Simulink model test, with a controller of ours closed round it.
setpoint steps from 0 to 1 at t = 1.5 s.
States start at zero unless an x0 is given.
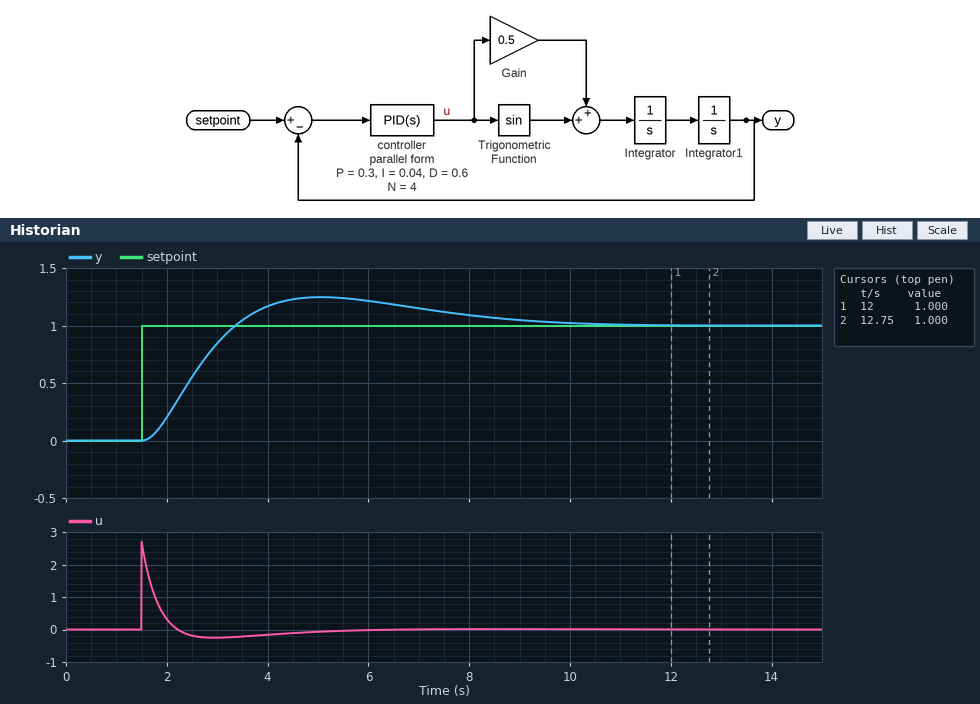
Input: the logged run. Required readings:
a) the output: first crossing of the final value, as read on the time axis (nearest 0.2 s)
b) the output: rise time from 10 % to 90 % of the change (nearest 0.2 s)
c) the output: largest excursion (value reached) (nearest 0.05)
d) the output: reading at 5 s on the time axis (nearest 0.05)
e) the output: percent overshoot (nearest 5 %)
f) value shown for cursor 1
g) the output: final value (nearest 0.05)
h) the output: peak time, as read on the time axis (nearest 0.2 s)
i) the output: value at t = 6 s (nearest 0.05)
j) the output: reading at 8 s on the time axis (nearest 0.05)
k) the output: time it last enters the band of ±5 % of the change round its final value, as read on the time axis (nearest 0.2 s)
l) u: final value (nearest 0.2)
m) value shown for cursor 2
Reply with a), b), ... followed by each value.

a) 3.4 s
b) 1.2 s
c) 1.25
d) 1.25
e) 25 %
f) 1.000
g) 1.00
h) 5.0 s
i) 1.20
j) 1.10
k) 9.0 s
l) 0.0
m) 1.000
